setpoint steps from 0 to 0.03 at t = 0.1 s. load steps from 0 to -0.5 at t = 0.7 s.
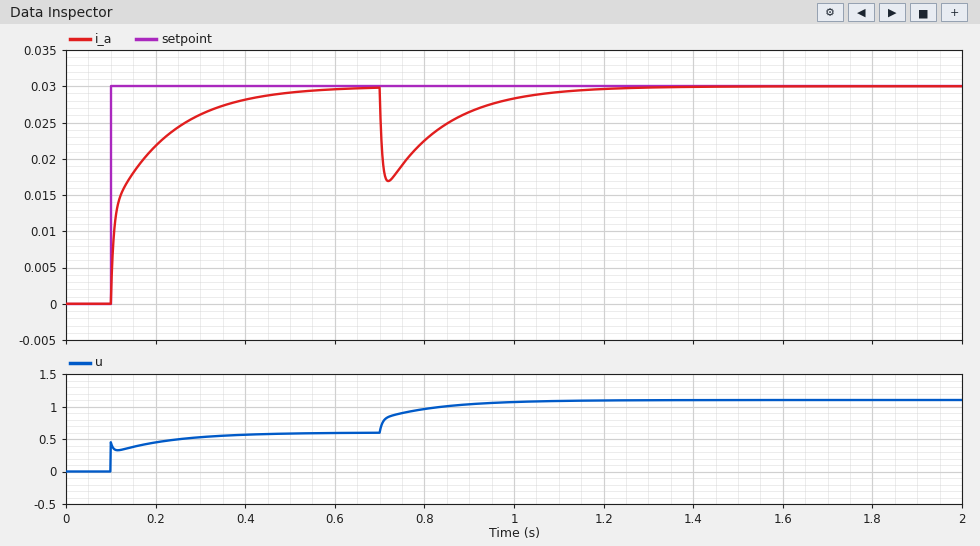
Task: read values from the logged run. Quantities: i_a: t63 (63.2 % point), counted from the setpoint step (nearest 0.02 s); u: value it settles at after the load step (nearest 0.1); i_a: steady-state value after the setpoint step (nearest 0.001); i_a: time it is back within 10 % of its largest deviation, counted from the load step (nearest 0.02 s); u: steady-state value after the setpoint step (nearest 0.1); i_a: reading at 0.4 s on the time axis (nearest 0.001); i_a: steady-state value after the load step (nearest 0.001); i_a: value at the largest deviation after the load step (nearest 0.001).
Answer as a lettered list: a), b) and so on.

a) 0.06 s
b) 1.1
c) 0.030
d) 0.34 s
e) 0.6
f) 0.028
g) 0.030
h) 0.017
